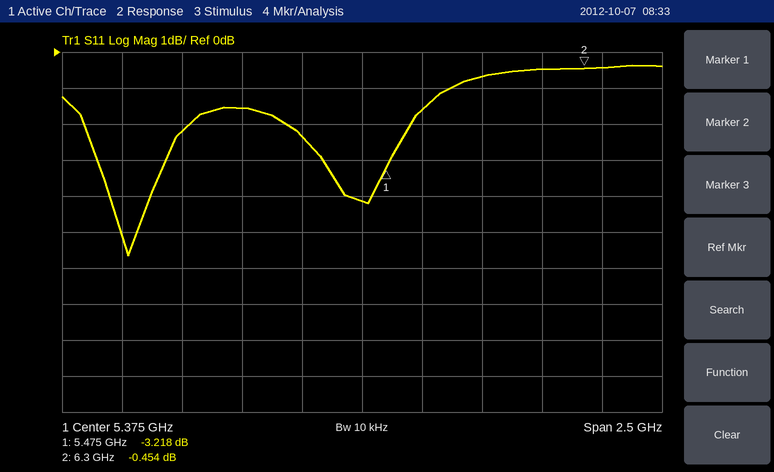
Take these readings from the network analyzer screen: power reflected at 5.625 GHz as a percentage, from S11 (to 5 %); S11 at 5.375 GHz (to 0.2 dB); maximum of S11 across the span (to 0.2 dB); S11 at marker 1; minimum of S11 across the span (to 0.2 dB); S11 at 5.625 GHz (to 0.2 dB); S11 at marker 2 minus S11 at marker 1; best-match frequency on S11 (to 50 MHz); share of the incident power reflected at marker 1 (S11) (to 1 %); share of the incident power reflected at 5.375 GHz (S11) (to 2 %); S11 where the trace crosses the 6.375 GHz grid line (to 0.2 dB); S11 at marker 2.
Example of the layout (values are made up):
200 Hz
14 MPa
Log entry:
70 %
-4.2 dB
-0.4 dB
-3.218 dB
-5.6 dB
-1.6 dB
2.764 dB
4.40 GHz
48 %
38 %
-0.4 dB
-0.454 dB
